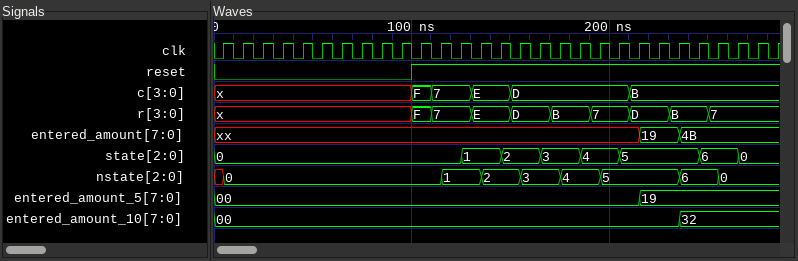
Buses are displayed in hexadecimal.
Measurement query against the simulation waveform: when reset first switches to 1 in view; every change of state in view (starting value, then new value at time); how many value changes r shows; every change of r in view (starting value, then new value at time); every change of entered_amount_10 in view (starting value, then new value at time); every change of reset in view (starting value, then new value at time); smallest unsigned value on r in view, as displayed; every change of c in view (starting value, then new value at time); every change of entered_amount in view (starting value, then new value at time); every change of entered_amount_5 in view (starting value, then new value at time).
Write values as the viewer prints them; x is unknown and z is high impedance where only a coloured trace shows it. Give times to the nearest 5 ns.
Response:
100 ns
0, 1 at 125 ns, 2 at 145 ns, 3 at 165 ns, 4 at 185 ns, 5 at 205 ns, 6 at 245 ns, 0 at 265 ns
9
x, F at 100 ns, 7 at 110 ns, E at 130 ns, D at 150 ns, B at 170 ns, 7 at 190 ns, D at 210 ns, B at 230 ns, 7 at 250 ns
00, 32 at 235 ns
0, 1 at 100 ns
7
x, F at 100 ns, 7 at 110 ns, E at 130 ns, D at 150 ns, B at 210 ns
xx, 19 at 215 ns, 4B at 235 ns
00, 19 at 215 ns
